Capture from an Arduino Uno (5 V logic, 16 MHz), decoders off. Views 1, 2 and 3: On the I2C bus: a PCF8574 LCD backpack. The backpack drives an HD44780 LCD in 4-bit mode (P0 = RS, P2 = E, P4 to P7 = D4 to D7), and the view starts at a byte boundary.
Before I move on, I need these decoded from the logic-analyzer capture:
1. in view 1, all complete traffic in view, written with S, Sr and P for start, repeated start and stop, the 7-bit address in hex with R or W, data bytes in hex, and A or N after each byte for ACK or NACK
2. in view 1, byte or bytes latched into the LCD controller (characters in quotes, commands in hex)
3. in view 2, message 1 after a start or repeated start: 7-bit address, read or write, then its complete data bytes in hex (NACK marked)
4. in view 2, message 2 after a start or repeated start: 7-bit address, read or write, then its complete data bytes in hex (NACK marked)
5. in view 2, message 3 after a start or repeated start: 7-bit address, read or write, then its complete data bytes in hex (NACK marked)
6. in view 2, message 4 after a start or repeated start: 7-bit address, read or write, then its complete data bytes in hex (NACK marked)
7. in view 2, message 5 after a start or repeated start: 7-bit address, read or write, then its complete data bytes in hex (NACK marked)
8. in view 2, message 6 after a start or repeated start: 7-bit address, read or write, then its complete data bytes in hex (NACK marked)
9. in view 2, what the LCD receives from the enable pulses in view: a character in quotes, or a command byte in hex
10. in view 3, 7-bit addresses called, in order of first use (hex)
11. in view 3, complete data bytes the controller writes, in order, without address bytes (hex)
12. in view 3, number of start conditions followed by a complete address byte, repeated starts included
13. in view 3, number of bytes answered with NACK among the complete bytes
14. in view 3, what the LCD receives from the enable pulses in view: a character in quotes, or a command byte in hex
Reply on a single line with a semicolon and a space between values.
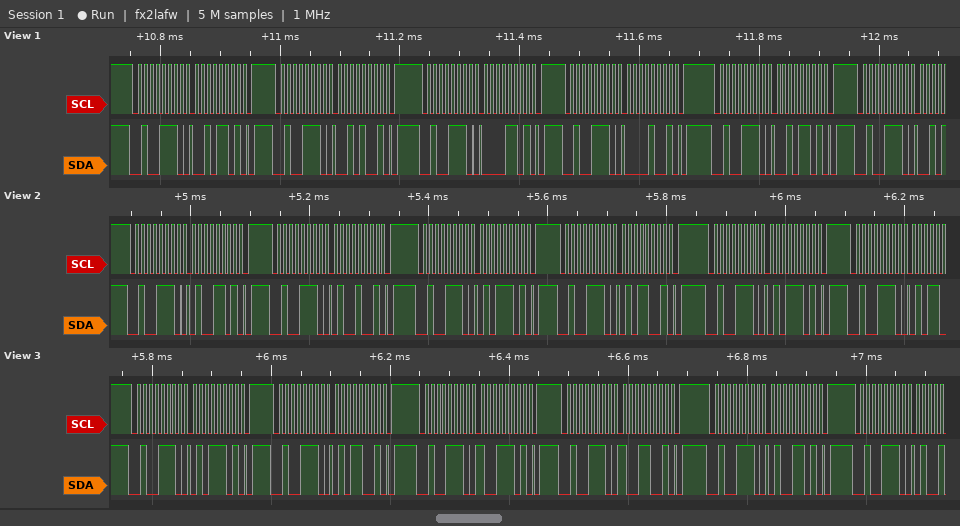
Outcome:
S 27W A 2D A P S 27W A 29 A P S 27W A 0D A P S 27W A 09 A P S 27W A 2D A P S 27W A; ' '; 0x27 write: 4D; 0x27 write: 49; 0x27 write: 5D; 0x27 write: 59; 0x27 write: 5D; 0x27 write; 'E'; 0x27; 5D 59 9D 99 4D; 6; 0; 'Y'
